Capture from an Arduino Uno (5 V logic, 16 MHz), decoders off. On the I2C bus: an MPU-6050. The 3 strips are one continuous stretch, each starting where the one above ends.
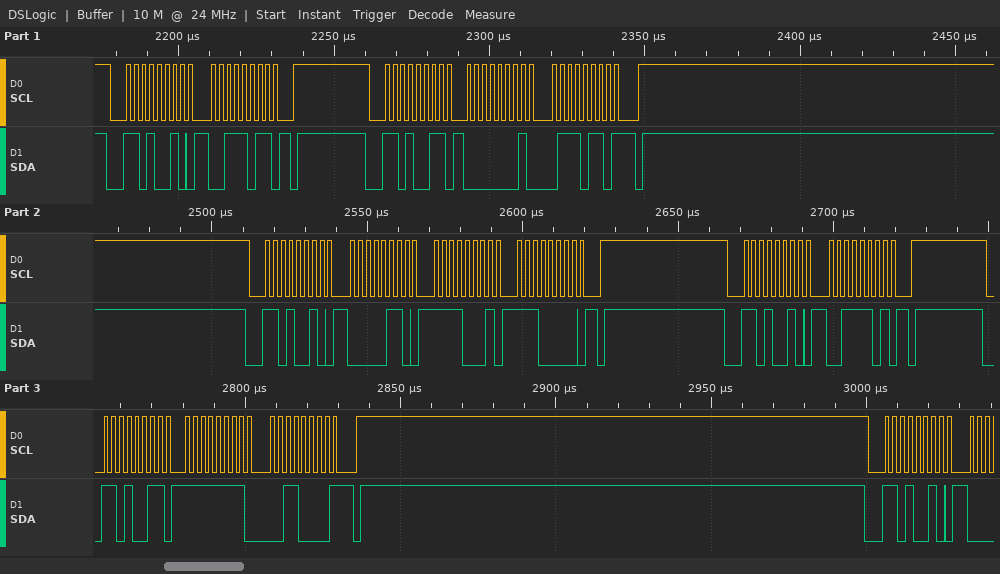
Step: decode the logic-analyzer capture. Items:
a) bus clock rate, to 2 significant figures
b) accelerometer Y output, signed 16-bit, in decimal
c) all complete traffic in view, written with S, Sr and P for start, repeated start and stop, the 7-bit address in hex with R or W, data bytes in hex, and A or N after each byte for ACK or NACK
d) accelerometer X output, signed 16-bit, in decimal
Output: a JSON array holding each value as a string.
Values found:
["400 kHz", "-208", "S 69W A 3B A P S 69R A 01 A 76 N P S 69W A 06 A F1 A E0 A P S 69W A 3D A P S 69R A FF A 30 N P S 69W A", "374"]
